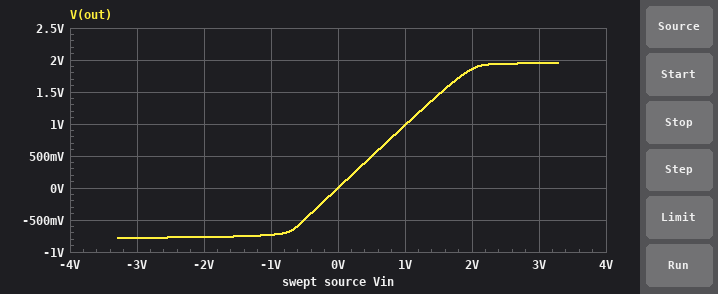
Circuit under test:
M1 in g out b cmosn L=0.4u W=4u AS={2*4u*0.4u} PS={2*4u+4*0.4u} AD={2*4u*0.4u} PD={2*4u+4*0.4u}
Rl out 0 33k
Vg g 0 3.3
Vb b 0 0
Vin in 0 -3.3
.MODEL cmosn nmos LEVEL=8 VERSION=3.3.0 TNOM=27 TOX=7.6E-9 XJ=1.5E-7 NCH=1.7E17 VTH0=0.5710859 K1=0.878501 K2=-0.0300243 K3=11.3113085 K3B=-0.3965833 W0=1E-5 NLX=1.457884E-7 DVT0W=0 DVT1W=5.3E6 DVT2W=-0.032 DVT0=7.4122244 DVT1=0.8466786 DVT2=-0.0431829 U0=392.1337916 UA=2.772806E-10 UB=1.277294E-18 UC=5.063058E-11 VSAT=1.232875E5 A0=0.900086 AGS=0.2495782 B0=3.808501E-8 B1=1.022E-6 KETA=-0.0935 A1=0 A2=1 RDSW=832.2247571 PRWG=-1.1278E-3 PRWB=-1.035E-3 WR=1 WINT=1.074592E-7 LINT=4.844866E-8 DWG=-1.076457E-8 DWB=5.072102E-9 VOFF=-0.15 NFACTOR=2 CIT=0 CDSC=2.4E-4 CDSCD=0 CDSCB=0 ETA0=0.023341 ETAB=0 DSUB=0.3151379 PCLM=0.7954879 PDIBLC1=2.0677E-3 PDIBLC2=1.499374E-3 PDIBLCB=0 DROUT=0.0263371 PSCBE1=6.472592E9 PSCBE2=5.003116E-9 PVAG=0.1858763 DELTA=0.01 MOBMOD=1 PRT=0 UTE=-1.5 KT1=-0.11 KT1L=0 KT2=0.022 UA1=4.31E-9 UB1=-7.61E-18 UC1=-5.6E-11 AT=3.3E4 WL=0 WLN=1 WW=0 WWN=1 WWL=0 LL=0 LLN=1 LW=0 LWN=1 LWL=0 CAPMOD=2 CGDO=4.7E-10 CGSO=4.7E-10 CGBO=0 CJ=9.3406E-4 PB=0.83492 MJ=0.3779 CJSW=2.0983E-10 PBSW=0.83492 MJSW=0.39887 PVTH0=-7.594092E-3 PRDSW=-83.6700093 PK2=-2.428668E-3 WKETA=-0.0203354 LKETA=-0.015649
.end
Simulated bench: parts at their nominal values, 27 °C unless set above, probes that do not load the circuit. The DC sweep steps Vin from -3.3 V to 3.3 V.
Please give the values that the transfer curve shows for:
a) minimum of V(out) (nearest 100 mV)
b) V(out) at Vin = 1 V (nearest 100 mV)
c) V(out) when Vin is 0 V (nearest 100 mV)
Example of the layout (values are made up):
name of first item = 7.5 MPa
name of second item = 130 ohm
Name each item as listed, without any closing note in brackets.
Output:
minimum of V(out) = -800 mV
V(out) at Vin = 1 V = 1.0 V
V(out) when Vin is 0 V = 0 V
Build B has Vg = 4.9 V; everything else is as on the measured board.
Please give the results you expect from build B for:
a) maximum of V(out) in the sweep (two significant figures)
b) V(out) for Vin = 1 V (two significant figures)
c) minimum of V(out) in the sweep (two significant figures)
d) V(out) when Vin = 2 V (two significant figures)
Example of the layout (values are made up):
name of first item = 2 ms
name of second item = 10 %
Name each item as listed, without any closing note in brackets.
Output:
maximum of V(out) in the sweep = 3.1 V
V(out) for Vin = 1 V = 990 mV
minimum of V(out) in the sweep = -780 mV
V(out) when Vin = 2 V = 2.0 V
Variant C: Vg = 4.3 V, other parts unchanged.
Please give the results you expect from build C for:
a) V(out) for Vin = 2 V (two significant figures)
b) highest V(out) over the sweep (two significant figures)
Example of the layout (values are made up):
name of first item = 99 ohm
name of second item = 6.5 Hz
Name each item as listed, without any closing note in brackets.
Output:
V(out) for Vin = 2 V = 2.0 V
highest V(out) over the sweep = 2.8 V
